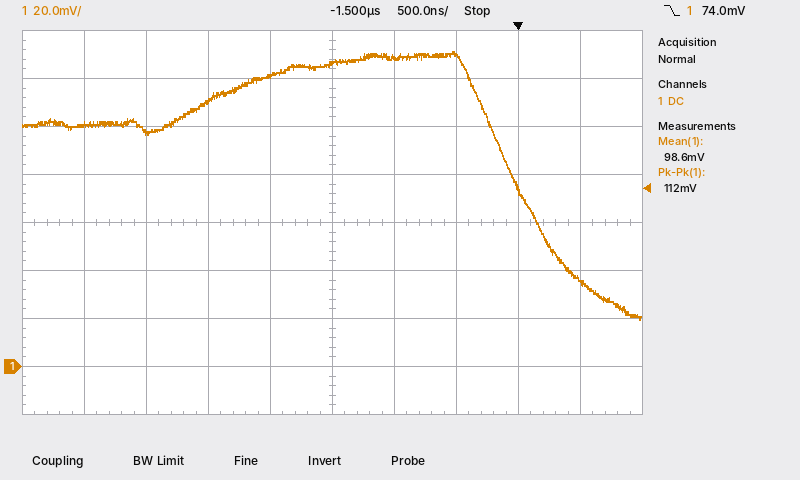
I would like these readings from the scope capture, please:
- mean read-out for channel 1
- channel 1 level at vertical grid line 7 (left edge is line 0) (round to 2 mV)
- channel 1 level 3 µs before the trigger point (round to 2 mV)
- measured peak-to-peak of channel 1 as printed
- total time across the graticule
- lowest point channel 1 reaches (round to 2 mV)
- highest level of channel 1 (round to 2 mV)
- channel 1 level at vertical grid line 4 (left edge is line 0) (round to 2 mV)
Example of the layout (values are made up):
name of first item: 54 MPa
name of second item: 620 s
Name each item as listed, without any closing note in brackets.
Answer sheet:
mean read-out for channel 1: 98.6 mV
channel 1 level at vertical grid line 7 (left edge is line 0): 130 mV
channel 1 level 3 µs before the trigger point: 98 mV
measured peak-to-peak of channel 1 as printed: 112 mV
total time across the graticule: 5 µs
lowest point channel 1 reaches: 20 mV
highest level of channel 1: 132 mV
channel 1 level at vertical grid line 4 (left edge is line 0): 122 mV
